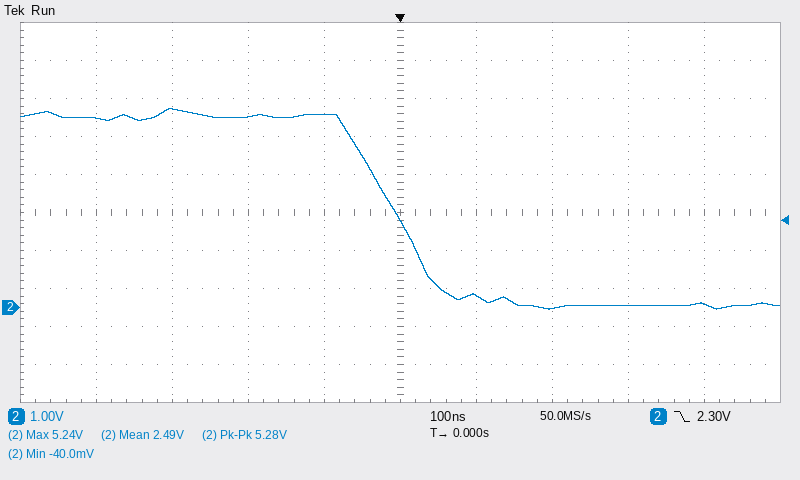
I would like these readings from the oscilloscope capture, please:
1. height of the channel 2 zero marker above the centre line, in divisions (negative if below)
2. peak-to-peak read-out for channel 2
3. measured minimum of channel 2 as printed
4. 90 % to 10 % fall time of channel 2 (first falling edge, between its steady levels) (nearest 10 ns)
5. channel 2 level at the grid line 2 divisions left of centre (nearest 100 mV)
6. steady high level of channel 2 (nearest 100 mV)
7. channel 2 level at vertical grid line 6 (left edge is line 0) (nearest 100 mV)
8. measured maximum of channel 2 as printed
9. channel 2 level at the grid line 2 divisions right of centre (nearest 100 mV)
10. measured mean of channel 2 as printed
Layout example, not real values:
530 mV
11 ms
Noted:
-2.5 div
5.28 V
-40.0 mV
120 ns
5.0 V
5.0 V
300 mV
5.24 V
0.0 V
2.49 V
